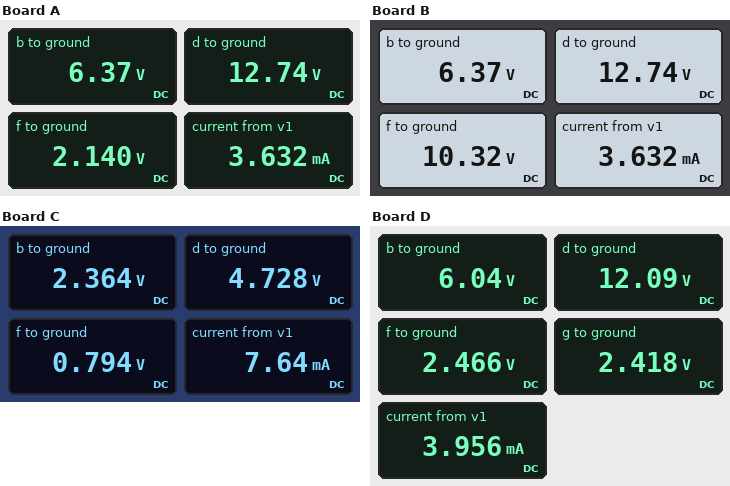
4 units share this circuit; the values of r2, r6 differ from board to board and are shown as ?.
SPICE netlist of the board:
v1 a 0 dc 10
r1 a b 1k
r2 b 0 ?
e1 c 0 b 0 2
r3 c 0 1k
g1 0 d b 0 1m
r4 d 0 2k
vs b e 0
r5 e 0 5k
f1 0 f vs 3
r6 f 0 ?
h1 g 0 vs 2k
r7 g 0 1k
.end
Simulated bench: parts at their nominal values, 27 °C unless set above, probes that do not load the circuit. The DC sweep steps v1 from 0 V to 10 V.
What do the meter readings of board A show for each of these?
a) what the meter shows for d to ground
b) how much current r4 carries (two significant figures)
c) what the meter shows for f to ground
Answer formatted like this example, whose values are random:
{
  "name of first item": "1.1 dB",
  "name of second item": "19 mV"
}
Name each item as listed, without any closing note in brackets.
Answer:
{
  "what the meter shows for d to ground": "12.74 V",
  "how much current r4 carries": "6.4 mA",
  "what the meter shows for f to ground": "2.140 V"
}
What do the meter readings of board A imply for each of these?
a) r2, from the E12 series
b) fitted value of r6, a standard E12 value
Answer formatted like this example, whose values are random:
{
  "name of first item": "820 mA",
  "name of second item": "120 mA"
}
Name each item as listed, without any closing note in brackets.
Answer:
{
  "r2, from the E12 series": "2.7 kΩ",
  "fitted value of r6, a standard E12 value": "560 Ω"
}
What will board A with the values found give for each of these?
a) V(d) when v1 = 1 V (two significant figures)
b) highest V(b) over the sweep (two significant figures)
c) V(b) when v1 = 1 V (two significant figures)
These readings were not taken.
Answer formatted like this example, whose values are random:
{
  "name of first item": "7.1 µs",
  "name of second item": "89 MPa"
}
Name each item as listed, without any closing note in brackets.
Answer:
{
  "V(d) when v1 = 1 V": "1.3 V",
  "highest V(b) over the sweep": "6.4 V",
  "V(b) when v1 = 1 V": "640 mV"
}
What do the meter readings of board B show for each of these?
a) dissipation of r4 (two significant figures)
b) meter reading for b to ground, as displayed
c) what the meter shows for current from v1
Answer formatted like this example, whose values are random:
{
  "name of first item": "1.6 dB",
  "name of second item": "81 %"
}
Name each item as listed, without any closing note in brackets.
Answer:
{
  "dissipation of r4": "81 mW",
  "meter reading for b to ground, as displayed": "6.37 V",
  "what the meter shows for current from v1": "3.632 mA"
}
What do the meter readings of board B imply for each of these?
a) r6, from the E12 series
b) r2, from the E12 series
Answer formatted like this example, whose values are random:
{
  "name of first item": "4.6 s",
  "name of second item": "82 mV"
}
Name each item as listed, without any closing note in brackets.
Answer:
{
  "r6, from the E12 series": "2.7 kΩ",
  "r2, from the E12 series": "2.7 kΩ"
}
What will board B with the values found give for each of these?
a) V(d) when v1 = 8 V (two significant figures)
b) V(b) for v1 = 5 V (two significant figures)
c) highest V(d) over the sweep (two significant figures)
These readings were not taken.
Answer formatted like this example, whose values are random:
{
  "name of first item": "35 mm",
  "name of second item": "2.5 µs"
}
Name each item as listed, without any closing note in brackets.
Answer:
{
  "V(d) when v1 = 8 V": "10 V",
  "V(b) for v1 = 5 V": "3.2 V",
  "highest V(d) over the sweep": "13 V"
}
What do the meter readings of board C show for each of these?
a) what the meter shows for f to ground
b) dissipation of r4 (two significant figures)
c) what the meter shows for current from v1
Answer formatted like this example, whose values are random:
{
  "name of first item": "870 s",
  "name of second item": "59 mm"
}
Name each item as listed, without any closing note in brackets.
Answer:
{
  "what the meter shows for f to ground": "0.794 V",
  "dissipation of r4": "11 mW",
  "what the meter shows for current from v1": "7.64 mA"
}
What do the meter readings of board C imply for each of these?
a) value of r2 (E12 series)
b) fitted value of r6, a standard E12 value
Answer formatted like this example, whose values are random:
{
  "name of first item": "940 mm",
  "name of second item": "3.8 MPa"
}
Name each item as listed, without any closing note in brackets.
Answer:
{
  "value of r2": "330 Ω",
  "fitted value of r6, a standard E12 value": "560 Ω"
}
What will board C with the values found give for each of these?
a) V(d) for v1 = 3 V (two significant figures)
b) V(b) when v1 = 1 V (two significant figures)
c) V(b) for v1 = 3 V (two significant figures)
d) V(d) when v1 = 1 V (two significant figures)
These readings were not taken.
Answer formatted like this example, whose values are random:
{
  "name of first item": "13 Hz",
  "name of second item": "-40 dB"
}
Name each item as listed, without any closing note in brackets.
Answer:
{
  "V(d) for v1 = 3 V": "1.4 V",
  "V(b) when v1 = 1 V": "240 mV",
  "V(b) for v1 = 3 V": "710 mV",
  "V(d) when v1 = 1 V": "470 mV"
}
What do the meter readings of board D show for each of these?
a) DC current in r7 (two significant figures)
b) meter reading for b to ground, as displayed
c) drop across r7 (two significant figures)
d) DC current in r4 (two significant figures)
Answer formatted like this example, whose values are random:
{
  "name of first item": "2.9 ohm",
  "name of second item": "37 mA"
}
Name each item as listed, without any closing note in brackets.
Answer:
{
  "DC current in r7": "2.4 mA",
  "meter reading for b to ground, as displayed": "6.04 V",
  "drop across r7": "2.4 V",
  "DC current in r4": "6.0 mA"
}
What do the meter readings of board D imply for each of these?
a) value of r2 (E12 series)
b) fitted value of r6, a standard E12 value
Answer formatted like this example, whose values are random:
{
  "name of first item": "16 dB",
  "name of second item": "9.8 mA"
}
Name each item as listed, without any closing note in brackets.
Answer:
{
  "value of r2": "2.2 kΩ",
  "fitted value of r6, a standard E12 value": "680 Ω"
}
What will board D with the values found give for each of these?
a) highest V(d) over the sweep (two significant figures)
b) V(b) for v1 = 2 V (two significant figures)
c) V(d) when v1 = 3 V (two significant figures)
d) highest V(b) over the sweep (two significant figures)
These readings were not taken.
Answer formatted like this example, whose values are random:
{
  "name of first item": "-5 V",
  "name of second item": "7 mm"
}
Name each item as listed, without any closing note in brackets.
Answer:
{
  "highest V(d) over the sweep": "12 V",
  "V(b) for v1 = 2 V": "1.2 V",
  "V(d) when v1 = 3 V": "3.6 V",
  "highest V(b) over the sweep": "6.0 V"
}
